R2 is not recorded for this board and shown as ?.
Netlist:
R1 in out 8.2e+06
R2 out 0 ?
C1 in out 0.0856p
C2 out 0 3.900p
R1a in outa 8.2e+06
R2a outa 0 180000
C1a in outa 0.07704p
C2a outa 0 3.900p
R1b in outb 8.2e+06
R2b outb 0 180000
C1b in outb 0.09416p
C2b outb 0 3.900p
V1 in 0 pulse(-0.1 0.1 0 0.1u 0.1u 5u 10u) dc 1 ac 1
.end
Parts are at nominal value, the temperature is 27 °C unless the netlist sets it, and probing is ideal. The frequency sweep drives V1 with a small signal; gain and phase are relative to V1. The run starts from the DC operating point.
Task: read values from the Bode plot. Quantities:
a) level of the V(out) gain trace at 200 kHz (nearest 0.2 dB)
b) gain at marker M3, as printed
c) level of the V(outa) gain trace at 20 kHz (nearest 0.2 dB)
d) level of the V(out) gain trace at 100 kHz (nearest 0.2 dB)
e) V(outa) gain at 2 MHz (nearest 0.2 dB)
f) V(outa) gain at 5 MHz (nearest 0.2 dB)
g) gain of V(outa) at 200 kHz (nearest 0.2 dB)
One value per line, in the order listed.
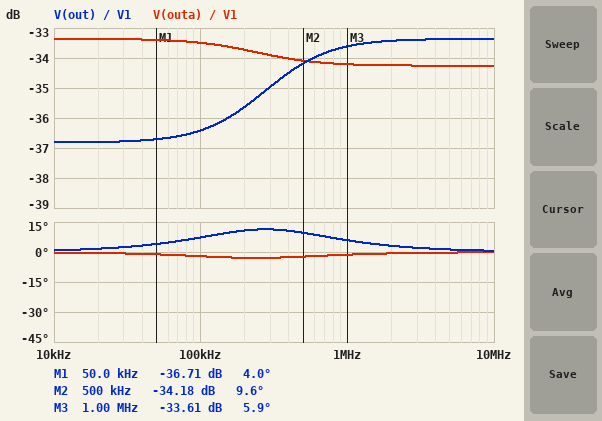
-35.6 dB
-33.61 dB
-33.4 dB
-36.4 dB
-34.2 dB
-34.2 dB
-33.8 dB
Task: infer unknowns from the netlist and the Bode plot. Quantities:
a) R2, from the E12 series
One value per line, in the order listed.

120 kΩ
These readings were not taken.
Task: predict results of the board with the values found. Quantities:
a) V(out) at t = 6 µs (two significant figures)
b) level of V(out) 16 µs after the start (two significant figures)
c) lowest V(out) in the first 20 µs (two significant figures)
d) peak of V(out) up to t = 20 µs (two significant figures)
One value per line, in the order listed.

-1.7 mV
-1.7 mV
-2.7 mV
2.7 mV
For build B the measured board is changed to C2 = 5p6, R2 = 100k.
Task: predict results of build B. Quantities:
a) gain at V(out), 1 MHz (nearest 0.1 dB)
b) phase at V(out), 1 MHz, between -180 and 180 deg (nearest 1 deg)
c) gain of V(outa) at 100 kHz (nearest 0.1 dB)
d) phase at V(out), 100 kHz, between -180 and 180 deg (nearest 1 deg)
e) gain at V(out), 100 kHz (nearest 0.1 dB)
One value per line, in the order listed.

-36.6 dB
3 deg
-33.5 dB
4 deg
-38.1 dB
